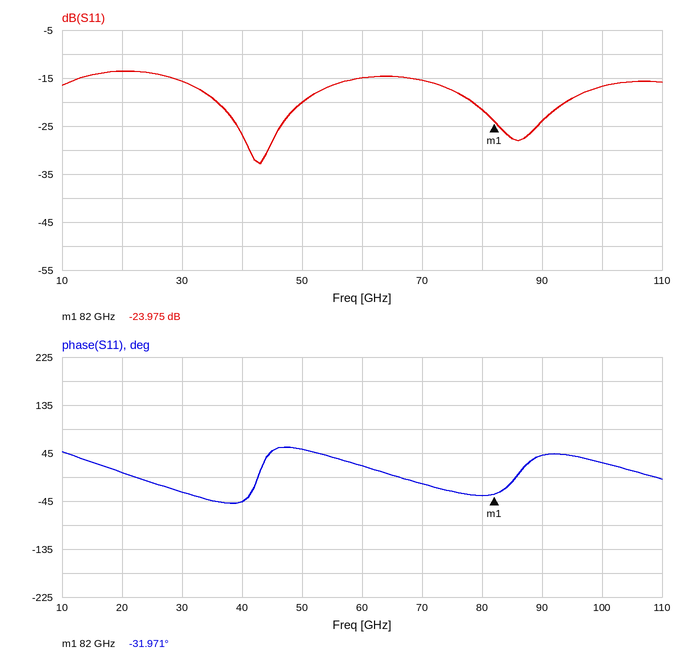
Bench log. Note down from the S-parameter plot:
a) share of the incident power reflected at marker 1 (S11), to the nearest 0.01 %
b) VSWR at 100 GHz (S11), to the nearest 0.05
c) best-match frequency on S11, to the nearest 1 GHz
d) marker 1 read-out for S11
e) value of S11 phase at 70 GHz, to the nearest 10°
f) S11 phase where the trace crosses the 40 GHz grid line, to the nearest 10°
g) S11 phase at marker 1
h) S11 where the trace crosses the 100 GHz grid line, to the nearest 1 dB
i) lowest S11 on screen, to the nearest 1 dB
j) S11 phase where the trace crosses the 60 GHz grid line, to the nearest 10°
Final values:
0.40 %
1.35
43 GHz
-23.975 dB
-10°
-50°
-31.971°
-17 dB
-33 dB
20°
